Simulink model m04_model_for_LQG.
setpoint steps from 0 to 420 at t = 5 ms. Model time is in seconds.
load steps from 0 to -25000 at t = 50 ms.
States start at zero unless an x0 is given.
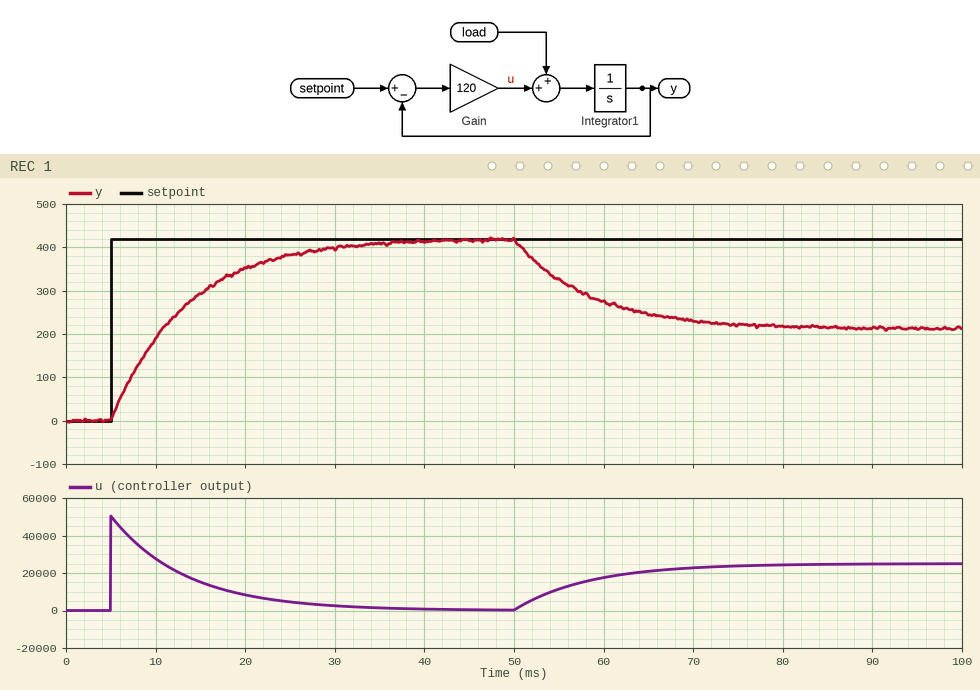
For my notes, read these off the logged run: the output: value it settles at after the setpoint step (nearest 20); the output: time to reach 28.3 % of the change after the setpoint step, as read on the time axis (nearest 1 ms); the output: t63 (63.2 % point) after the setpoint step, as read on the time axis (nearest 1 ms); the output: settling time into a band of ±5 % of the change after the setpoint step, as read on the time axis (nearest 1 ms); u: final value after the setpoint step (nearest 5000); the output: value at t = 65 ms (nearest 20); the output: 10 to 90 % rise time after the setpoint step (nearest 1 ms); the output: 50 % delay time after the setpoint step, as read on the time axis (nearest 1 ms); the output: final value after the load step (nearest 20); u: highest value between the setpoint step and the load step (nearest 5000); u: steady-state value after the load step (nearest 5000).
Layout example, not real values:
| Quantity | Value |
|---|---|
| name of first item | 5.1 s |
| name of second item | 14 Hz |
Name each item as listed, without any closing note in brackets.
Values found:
| Quantity | Value |
|---|---|
| the output: value it settles at after the setpoint step | 420 |
| the output: time to reach 28.3 % of the change after the setpoint step, as read on the time axis | 8 ms |
| the output: t63 (63.2 % point) after the setpoint step, as read on the time axis | 13 ms |
| the output: settling time into a band of ±5 % of the change after the setpoint step, as read on the time axis | 30 ms |
| u: final value after the setpoint step | 0 |
| the output: value at t = 65 ms | 240 |
| the output: 10 to 90 % rise time after the setpoint step | 18 ms |
| the output: 50 % delay time after the setpoint step, as read on the time axis | 11 ms |
| the output: final value after the load step | 220 |
| u: highest value between the setpoint step and the load step | 50000 |
| u: steady-state value after the load step | 25000 |
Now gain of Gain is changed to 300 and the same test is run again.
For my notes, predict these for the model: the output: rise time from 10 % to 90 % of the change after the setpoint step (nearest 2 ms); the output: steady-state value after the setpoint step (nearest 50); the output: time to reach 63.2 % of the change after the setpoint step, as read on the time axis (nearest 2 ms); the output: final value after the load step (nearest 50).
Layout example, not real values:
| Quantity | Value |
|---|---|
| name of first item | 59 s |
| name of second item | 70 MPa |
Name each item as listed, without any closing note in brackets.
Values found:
| Quantity | Value |
|---|---|
| the output: rise time from 10 % to 90 % of the change after the setpoint step | 8 ms |
| the output: steady-state value after the setpoint step | 400 |
| the output: time to reach 63.2 % of the change after the setpoint step, as read on the time axis | 8 ms |
| the output: final value after the load step | 350 |
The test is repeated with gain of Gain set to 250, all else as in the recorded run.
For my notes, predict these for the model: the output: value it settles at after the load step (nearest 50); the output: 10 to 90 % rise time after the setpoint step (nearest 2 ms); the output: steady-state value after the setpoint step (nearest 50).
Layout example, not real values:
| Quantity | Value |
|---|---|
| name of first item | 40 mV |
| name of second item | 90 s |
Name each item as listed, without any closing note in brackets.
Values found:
| Quantity | Value |
|---|---|
| the output: value it settles at after the load step | 300 |
| the output: 10 to 90 % rise time after the setpoint step | 8 ms |
| the output: steady-state value after the setpoint step | 400 |
